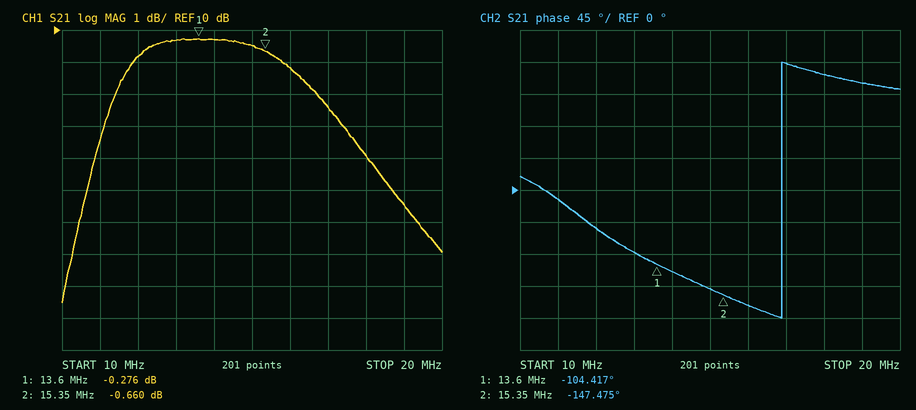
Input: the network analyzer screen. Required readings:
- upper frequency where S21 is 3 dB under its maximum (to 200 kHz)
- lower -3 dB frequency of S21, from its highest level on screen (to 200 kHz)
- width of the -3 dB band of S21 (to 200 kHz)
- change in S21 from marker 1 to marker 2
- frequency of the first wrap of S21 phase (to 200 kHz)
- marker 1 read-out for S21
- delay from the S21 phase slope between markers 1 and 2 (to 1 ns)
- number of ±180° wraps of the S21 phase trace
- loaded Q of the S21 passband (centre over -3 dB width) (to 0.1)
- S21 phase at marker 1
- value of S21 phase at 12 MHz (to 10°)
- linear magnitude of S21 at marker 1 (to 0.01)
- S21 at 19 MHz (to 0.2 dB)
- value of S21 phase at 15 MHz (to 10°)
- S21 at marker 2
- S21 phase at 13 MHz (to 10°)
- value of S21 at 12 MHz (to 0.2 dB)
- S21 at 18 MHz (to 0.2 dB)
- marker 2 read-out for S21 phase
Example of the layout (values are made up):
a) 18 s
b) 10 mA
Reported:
a) 17.6 MHz
b) 11.0 MHz
c) 6.6 MHz
d) -0.384 dB
e) 16.8 MHz
f) -0.276 dB
g) 68 ns
h) 1
i) 2.2
j) -104.417°
k) -50°
l) 0.97
m) -5.4 dB
n) -140°
o) -0.660 dB
p) -90°
q) -0.8 dB
r) -4.0 dB
s) -147.475°
